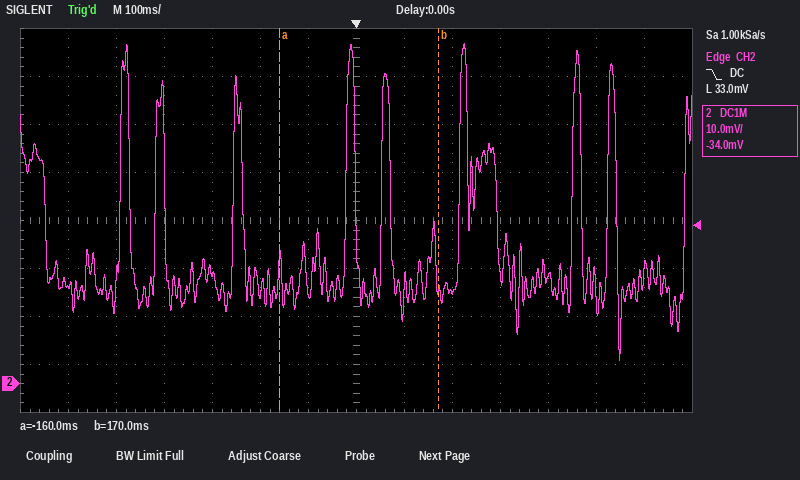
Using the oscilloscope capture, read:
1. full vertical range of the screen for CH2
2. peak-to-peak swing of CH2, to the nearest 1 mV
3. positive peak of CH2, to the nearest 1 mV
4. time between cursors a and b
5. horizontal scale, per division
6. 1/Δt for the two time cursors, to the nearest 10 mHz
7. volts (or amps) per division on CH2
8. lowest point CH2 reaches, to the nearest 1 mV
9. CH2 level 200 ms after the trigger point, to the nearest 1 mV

80 mV
66 mV
71 mV
330 ms
100 ms
3.03 Hz
10 mV
5 mV
19 mV
